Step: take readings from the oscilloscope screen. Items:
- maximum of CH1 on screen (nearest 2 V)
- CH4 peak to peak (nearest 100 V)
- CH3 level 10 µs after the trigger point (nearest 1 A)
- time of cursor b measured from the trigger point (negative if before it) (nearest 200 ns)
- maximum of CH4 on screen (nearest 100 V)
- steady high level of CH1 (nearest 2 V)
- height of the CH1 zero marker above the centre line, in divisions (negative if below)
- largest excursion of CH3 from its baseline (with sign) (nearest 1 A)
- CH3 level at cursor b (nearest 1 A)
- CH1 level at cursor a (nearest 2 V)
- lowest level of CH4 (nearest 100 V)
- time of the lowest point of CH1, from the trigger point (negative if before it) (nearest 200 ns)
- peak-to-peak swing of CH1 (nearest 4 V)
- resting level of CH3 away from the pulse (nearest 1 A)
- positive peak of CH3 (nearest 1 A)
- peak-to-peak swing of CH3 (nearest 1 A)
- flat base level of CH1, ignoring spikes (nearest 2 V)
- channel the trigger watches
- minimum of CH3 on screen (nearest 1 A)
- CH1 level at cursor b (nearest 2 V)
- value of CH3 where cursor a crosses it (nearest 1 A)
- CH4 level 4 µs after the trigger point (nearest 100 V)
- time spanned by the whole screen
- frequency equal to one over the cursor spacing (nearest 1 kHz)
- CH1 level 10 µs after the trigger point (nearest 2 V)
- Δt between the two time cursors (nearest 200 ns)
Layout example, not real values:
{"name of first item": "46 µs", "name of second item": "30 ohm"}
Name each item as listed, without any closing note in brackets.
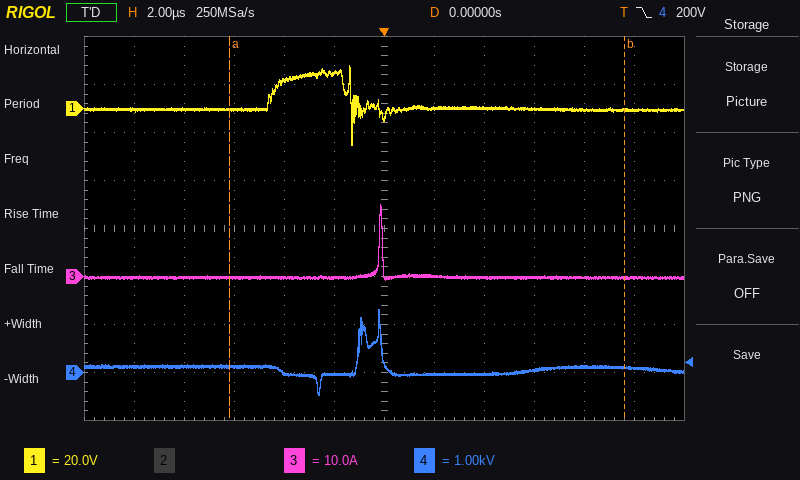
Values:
{"maximum of CH1 on screen": "18 V", "CH4 peak to peak": "1.8 kV", "CH3 level 10 µs after the trigger point": "0 A", "time of cursor b measured from the trigger point (negative if before it)": "+9.6 µs", "maximum of CH4 on screen": "1.3 kV", "steady high level of CH1": "14 V", "height of the CH1 zero marker above the centre line, in divisions": "+2.5 div", "largest excursion of CH3 from its baseline (with sign)": "+15 A", "CH3 level at cursor b": "0 A", "CH1 level at cursor a": "0 V", "lowest level of CH4": "-500 V", "time of the lowest point of CH1, from the trigger point (negative if before it)": "-1.2 µs", "peak-to-peak swing of CH1": "32 V", "resting level of CH3 away from the pulse": "0 A", "positive peak of CH3": "15 A", "peak-to-peak swing of CH3": "16 A", "flat base level of CH1, ignoring spikes": "0 V", "channel the trigger watches": "CH4", "minimum of CH3 on screen": "-1 A", "CH1 level at cursor b": "0 V", "value of CH3 where cursor a crosses it": "0 A", "CH4 level 4 µs after the trigger point": "0.0 kV", "time spanned by the whole screen": "24 µs", "frequency equal to one over the cursor spacing": "63 kHz", "CH1 level 10 µs after the trigger point": "0 V", "Δt between the two time cursors": "15.8 µs"}
